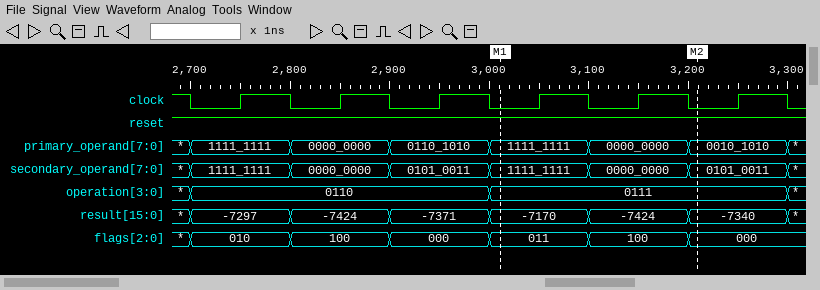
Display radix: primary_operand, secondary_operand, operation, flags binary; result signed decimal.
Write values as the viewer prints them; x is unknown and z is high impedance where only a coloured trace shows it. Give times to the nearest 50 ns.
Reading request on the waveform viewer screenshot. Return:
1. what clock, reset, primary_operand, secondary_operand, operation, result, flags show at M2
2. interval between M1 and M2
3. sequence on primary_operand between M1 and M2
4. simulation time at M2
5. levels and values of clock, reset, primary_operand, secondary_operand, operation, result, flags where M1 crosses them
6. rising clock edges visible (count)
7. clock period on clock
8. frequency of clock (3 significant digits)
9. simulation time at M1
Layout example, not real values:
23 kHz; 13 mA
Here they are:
clock=0, reset=1, primary_operand=0010_1010, secondary_operand=0101_0011, operation=0111, result=-7340, flags=000; 200 ns; 1111_1111, 0000_0000, 0010_1010; 3200 ns; clock=0, reset=1, primary_operand=1111_1111, secondary_operand=1111_1111, operation=0111, result=-7170, flags=011; 6; 100 ns; 10.0 MHz; 3000 ns
